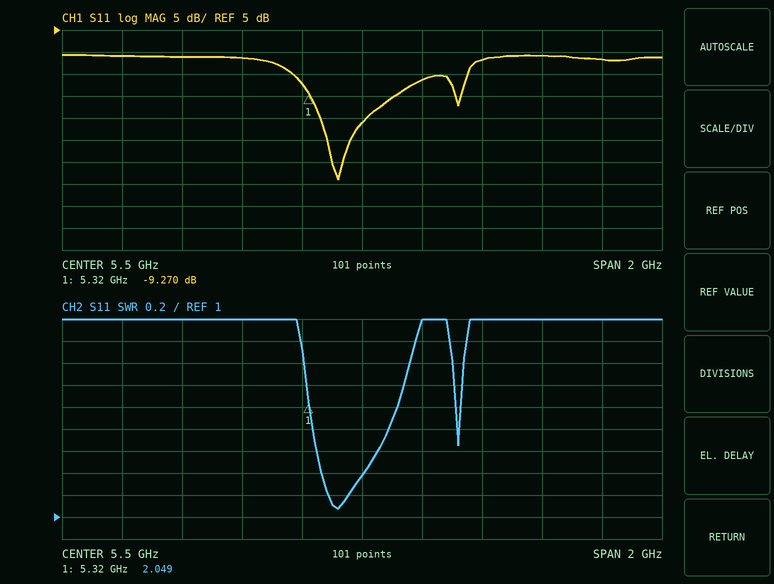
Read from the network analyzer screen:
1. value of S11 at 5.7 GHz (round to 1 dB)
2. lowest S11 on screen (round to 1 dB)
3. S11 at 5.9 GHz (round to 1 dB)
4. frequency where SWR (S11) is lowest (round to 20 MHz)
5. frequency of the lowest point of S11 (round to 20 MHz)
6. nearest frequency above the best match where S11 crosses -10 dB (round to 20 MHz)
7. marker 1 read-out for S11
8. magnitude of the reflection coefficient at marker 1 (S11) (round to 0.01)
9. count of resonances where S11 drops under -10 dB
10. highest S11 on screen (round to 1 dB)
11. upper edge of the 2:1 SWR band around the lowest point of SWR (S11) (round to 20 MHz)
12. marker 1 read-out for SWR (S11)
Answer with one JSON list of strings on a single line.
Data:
["-6 dB", "-29 dB", "-2 dB", "5.42 GHz", "5.42 GHz", "5.60 GHz", "-9.270 dB", "0.34", "2", "-1 dB", "5.62 GHz", "2.049"]
